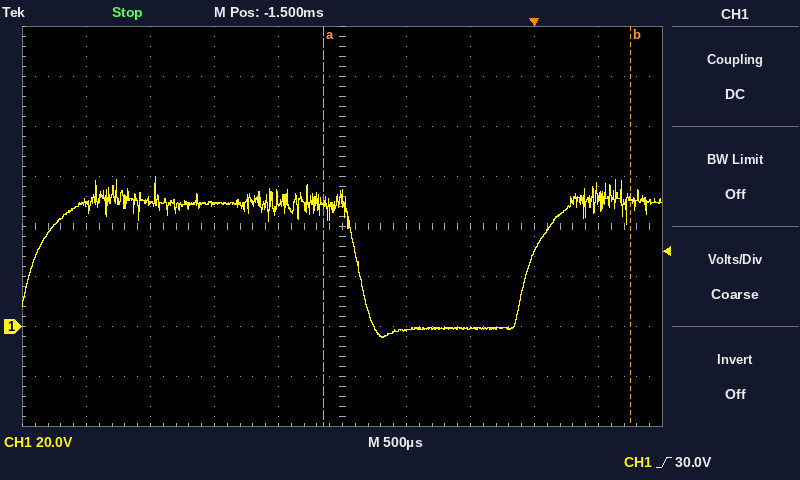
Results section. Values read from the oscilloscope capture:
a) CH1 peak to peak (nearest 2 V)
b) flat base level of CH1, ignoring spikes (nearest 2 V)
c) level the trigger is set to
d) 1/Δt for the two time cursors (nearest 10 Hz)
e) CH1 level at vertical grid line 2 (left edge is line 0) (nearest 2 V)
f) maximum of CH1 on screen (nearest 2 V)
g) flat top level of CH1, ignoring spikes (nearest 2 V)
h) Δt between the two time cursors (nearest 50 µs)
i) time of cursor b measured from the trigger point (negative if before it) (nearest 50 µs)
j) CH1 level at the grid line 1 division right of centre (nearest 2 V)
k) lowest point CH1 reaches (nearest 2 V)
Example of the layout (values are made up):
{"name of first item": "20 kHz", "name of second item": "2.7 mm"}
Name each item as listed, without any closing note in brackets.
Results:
{"CH1 peak to peak": "64 V", "flat base level of CH1, ignoring spikes": "0 V", "level the trigger is set to": "30.0 V", "1/Δt for the two time cursors": "420 Hz", "CH1 level at vertical grid line 2 (left edge is line 0)": "50 V", "maximum of CH1 on screen": "60 V", "flat top level of CH1, ignoring spikes": "50 V", "Δt between the two time cursors": "2.40 ms", "time of cursor b measured from the trigger point (negative if before it)": "+750 µs", "CH1 level at the grid line 1 division right of centre": "-2 V", "lowest point CH1 reaches": "-4 V"}
